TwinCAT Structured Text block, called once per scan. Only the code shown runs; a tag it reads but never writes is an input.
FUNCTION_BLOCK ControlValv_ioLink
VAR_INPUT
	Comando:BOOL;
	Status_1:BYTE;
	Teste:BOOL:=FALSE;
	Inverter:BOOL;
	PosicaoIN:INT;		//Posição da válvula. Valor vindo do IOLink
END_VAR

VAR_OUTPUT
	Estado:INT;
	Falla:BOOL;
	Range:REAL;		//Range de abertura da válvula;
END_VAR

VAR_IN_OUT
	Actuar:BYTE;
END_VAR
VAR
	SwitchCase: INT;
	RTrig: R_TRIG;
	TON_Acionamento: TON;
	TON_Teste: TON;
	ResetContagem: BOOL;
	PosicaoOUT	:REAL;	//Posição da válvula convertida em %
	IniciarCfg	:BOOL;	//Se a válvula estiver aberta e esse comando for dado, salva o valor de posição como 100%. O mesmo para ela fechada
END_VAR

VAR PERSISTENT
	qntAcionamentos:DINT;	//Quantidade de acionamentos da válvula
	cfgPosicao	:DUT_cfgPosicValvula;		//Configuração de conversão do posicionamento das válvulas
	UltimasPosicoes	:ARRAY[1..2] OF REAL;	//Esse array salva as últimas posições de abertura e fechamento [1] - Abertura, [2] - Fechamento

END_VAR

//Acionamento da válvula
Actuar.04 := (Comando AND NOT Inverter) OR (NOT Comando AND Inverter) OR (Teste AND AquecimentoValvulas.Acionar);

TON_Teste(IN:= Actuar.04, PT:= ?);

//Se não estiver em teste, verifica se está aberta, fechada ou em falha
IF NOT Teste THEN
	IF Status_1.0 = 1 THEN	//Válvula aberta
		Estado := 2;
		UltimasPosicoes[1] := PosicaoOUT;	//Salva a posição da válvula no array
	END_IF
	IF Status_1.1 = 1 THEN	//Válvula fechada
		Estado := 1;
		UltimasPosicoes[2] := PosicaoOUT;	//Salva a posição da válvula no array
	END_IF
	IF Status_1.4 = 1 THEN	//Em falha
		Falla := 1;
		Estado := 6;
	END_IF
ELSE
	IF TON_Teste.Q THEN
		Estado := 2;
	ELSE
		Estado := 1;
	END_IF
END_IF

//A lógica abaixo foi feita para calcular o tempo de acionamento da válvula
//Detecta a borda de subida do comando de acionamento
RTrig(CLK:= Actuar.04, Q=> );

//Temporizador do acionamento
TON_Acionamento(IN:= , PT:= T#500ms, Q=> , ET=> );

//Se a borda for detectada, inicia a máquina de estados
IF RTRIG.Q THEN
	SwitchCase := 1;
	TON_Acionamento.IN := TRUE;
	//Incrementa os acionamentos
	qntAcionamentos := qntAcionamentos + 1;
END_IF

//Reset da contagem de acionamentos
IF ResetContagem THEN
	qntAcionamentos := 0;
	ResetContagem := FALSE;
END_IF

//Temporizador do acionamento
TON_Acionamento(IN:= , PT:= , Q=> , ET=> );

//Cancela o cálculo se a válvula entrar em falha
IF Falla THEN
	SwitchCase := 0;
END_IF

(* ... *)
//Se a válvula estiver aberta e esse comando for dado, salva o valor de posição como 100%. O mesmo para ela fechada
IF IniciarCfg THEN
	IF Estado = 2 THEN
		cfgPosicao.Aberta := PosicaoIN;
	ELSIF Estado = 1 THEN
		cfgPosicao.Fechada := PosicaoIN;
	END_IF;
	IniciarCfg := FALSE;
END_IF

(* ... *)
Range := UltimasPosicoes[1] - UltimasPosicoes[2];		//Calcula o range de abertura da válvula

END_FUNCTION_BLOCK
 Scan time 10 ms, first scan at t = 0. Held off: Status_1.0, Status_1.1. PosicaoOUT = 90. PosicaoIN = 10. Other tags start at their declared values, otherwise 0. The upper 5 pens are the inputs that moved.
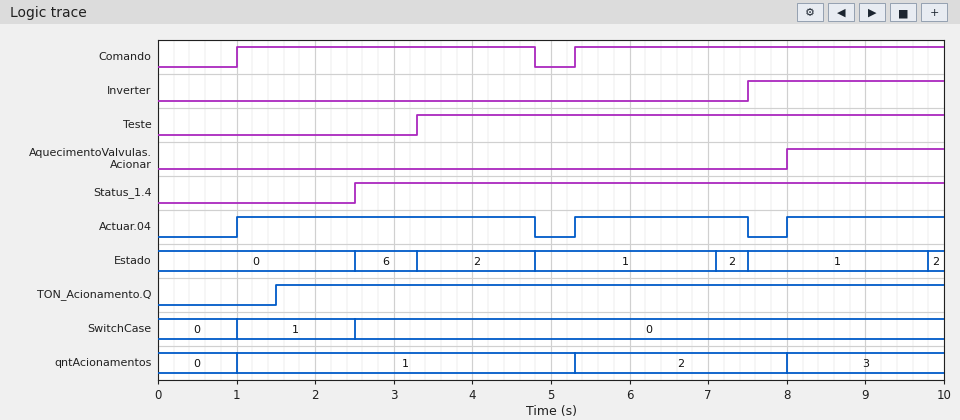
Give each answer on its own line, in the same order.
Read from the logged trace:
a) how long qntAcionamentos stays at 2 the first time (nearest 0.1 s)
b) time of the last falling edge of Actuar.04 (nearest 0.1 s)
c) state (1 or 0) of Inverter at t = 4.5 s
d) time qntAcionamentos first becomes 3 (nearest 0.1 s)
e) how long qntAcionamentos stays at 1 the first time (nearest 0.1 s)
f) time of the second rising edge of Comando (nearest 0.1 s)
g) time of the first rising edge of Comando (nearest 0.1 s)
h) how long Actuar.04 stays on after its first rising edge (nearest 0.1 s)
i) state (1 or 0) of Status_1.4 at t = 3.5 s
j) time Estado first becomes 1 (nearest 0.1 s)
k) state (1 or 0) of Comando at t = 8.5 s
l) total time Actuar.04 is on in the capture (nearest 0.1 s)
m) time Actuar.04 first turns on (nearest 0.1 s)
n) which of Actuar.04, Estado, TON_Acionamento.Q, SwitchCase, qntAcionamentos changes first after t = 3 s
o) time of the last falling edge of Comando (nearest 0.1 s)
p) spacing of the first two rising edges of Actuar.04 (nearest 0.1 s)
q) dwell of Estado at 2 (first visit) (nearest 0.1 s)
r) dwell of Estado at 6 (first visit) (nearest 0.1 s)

2.7 s
7.5 s
0
8.0 s
4.3 s
5.3 s
1.0 s
3.8 s
1
4.8 s
1
8.0 s
1.0 s
Estado
4.8 s
4.3 s
1.5 s
0.8 s
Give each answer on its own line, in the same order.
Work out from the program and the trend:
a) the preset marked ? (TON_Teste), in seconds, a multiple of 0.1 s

1.8 s
